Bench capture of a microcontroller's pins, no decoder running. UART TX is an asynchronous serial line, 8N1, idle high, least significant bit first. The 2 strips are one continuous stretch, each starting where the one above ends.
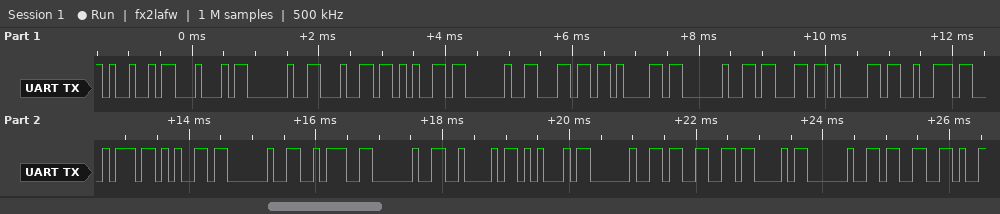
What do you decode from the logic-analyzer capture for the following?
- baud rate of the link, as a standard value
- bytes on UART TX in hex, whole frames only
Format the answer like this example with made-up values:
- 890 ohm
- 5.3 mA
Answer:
- 9600 baud
- 49 44 20 64 65 20 6C 61 20 63 61 72 74 65 20 3A 20 42 45 20 33 43 20 33
